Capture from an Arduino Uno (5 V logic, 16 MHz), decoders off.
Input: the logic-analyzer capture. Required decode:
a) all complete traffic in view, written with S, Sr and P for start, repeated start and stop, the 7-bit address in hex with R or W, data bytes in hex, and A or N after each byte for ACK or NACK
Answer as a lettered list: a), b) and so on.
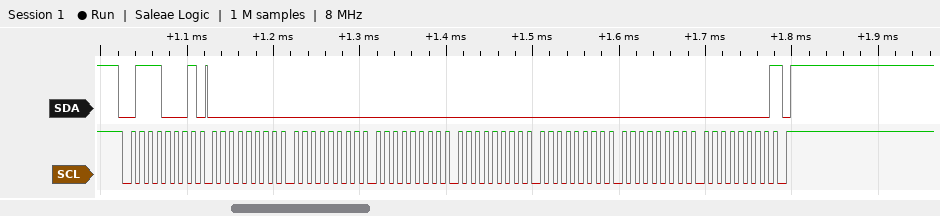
a) S 38R A 00 A 00 A 00 A 00 A 00 A 00 A 00 N P
